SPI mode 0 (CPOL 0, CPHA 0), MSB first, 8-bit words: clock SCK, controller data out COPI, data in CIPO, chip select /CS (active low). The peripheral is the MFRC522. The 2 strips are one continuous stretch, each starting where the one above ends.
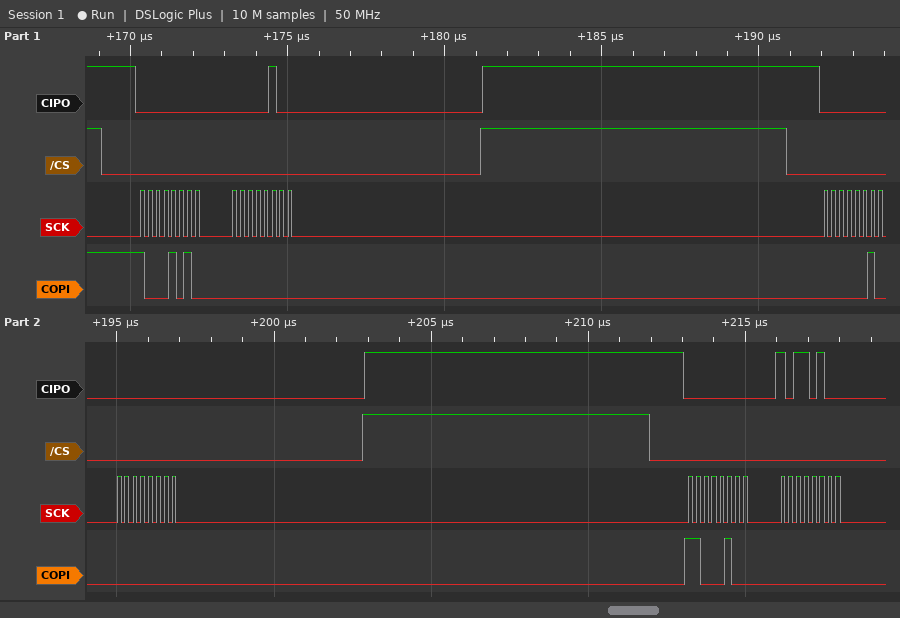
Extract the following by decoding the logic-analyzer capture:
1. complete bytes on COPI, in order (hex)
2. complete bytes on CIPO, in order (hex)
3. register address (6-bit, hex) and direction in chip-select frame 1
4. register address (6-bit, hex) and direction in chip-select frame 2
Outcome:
8A 00 02 00 C4 00
00 04 00 00 00 B4
0x05 read
0x01 write
